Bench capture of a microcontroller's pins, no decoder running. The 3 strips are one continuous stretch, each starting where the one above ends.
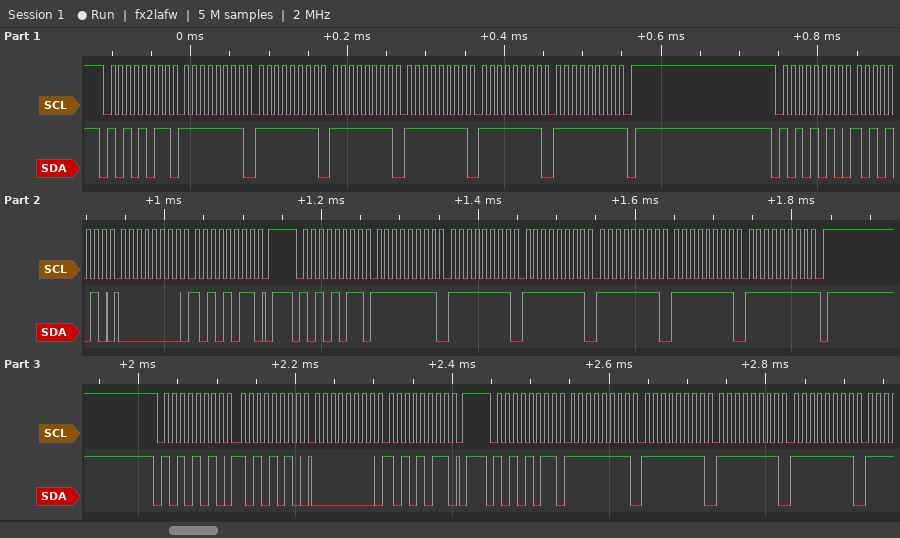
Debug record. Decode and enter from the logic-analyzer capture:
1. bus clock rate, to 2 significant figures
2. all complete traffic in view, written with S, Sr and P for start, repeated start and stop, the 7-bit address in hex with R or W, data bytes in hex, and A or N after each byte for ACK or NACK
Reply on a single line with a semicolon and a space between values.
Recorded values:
100 kHz; S 55R A FF A FF A FF A FF A FF A FF N P S 55W A AA A 00 A AB A P S 55R A FF A FF A FF A FF A FF A FF N P S 55W A AA A 00 A AB A P S 55R A FF A FF A FF A FF A
